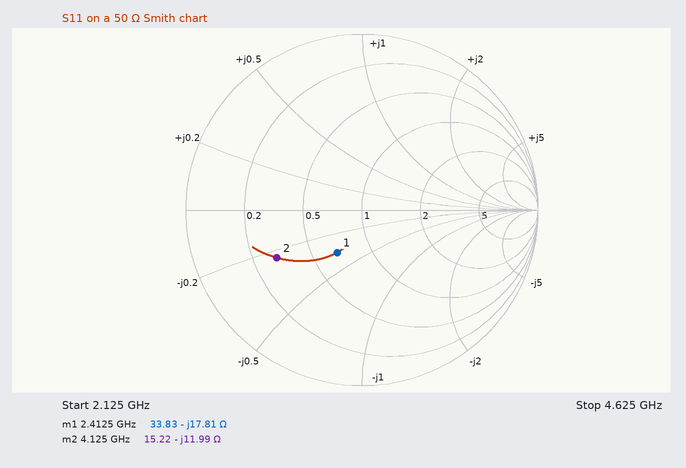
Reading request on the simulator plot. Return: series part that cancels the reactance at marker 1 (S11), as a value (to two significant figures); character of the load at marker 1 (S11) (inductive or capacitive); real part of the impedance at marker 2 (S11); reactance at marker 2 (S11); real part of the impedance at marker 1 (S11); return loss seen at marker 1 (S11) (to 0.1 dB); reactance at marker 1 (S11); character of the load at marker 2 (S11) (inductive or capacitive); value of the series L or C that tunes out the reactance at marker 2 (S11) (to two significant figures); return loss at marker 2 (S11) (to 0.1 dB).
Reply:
1.2 nH
capacitive
15.22 Ω
-11.99 Ω
33.83 Ω
11.0 dB
-17.81 Ω
capacitive
460 pH
5.1 dB
